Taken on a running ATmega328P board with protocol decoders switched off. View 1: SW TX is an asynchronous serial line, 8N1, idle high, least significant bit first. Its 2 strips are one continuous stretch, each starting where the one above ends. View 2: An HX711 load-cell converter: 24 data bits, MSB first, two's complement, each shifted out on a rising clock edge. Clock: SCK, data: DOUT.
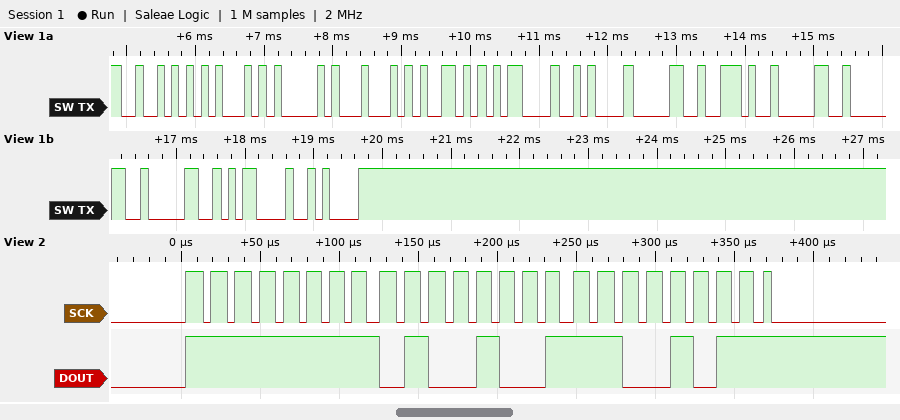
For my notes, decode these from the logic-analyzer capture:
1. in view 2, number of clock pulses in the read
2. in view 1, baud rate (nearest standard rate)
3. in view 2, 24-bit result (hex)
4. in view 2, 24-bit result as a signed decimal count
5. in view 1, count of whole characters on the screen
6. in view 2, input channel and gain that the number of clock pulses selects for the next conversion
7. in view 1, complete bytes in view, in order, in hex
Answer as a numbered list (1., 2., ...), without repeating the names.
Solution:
1. 25
2. 9600 baud
3. 0xFF49CB
4. -46645
5. 14
6. channel A, gain 128
7. 52 45 41 44 59 0D 0A 30 2E 30 30 30 0D 0A
